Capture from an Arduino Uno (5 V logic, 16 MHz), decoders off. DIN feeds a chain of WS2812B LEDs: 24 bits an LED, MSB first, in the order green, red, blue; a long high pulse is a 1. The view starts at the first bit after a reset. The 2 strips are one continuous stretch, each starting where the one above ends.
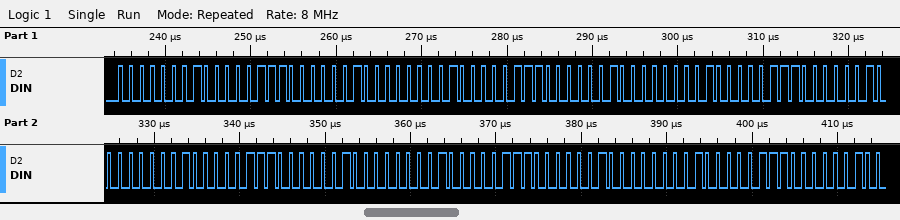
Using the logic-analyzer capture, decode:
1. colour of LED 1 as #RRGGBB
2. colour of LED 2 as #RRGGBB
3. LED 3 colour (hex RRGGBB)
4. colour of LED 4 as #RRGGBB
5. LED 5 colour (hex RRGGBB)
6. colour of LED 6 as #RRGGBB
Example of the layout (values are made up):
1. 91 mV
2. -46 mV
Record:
1. #070102
2. #070102
3. #070102
4. #070102
5. #070102
6. #070102
